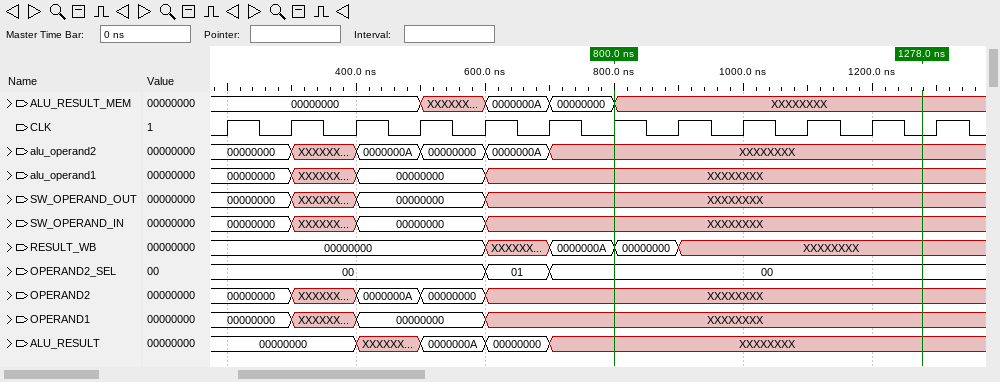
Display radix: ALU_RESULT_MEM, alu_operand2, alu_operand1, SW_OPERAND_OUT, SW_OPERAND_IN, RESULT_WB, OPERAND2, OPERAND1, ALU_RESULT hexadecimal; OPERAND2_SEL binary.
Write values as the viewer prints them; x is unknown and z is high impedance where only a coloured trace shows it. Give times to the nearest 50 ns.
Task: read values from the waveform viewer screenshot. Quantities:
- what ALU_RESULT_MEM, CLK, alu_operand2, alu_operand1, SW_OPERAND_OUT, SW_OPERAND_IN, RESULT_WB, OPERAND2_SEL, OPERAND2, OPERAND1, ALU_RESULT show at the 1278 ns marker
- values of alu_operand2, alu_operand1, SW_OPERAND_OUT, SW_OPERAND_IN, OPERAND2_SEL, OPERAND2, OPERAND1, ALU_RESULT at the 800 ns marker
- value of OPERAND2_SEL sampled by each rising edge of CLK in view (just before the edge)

ALU_RESULT_MEM=XXXXXXXX, CLK=0, alu_operand2=XXXXXXXX, alu_operand1=XXXXXXXX, SW_OPERAND_OUT=XXXXXXXX, SW_OPERAND_IN=XXXXXXXX, RESULT_WB=XXXXXXXX, OPERAND2_SEL=00, OPERAND2=XXXXXXXX, OPERAND1=XXXXXXXX, ALU_RESULT=XXXXXXXX
alu_operand2=XXXXXXXX, alu_operand1=XXXXXXXX, SW_OPERAND_OUT=XXXXXXXX, SW_OPERAND_IN=XXXXXXXX, OPERAND2_SEL=00, OPERAND2=XXXXXXXX, OPERAND1=XXXXXXXX, ALU_RESULT=XXXXXXXX
00, 00, 00, 00, 00, 01, 00, 00, 00, 00, 00, 00
